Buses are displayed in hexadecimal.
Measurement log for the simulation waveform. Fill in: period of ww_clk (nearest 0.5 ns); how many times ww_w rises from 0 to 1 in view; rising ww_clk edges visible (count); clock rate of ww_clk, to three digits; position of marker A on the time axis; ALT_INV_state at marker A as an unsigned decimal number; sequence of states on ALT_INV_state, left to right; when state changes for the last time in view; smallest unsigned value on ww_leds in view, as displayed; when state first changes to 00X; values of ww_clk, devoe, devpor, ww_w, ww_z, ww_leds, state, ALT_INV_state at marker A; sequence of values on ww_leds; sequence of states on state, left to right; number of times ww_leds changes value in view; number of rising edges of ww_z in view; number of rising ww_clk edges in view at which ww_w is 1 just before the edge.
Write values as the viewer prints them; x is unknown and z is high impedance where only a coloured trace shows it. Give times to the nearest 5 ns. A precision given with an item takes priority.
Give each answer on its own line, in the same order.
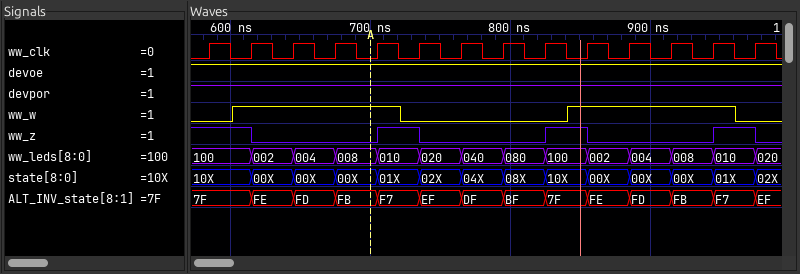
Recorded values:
30 ns
2
14
33.3 MHz
700 ns
251
7F, FE, FD, FB, F7, EF, DF, BF, 7F, FE, FD, FB, F7, EF
975 ns
002
615 ns
ww_clk=0, devoe=1, devpor=1, ww_w=1, ww_z=0, ww_leds=008, state=00X, ALT_INV_state=FB
100, 002, 004, 008, 010, 020, 040, 080, 100, 002, 004, 008, 010, 020
10X, 00X, 00X, 00X, 01X, 02X, 04X, 08X, 10X, 00X, 00X, 00X, 01X, 02X
13
3
8
